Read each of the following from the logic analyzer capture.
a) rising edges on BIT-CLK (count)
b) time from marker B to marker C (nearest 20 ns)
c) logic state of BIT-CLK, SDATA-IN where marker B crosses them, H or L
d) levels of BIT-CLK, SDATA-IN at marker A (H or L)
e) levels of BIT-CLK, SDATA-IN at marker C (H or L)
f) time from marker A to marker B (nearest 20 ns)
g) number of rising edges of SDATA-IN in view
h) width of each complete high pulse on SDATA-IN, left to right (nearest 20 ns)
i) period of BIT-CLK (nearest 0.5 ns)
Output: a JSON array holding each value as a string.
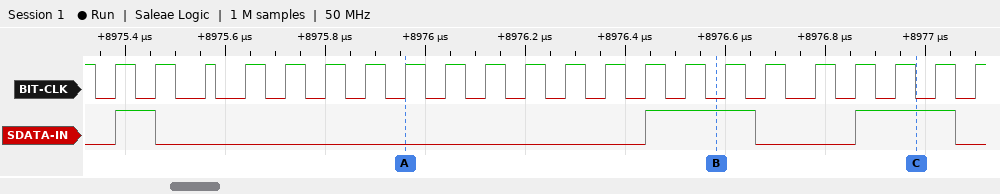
["22", "400 ns", "BIT-CLK=L, SDATA-IN=H", "BIT-CLK=H, SDATA-IN=L", "BIT-CLK=L, SDATA-IN=H", "620 ns", "3", "80 ns, 220 ns, 200 ns", "82 ns"]
